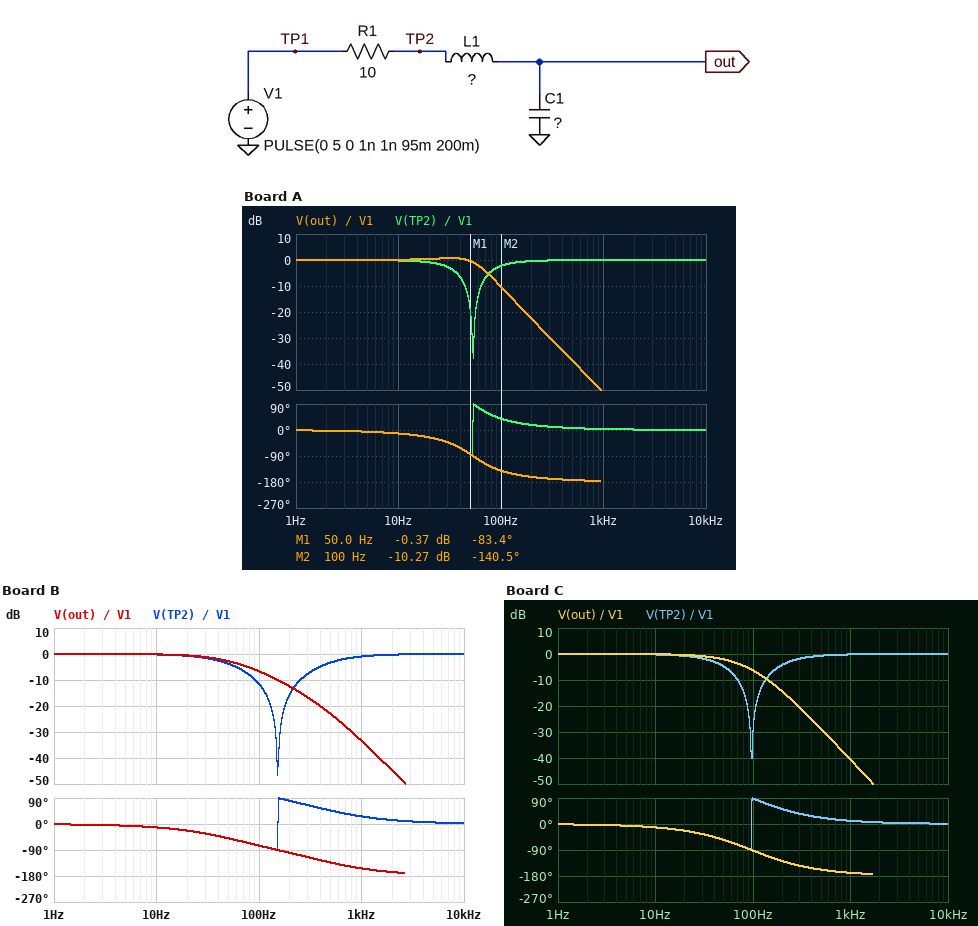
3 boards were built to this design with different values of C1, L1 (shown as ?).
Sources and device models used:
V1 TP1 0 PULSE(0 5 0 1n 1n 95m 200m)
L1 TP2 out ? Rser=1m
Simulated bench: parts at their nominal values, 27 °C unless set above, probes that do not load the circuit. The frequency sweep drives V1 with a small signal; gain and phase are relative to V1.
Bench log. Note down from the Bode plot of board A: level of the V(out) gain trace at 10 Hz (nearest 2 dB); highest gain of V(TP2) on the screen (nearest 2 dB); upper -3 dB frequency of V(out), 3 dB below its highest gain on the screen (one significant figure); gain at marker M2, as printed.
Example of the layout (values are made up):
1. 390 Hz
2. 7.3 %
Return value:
1. 0 dB
2. 0 dB
3. 60 Hz
4. -10.27 dB
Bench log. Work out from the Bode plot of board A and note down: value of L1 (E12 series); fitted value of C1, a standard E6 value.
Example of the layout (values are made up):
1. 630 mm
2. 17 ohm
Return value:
1. 27 mH
2. 330 µF
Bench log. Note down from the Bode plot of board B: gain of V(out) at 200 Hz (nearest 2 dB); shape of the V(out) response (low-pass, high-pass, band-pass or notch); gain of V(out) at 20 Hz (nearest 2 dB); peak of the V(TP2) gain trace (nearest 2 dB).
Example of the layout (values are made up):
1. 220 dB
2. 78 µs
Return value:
1. -12 dB
2. low-pass
3. 0 dB
4. 0 dB
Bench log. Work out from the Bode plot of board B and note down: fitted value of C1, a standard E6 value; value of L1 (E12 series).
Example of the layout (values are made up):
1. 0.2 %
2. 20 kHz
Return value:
1. 330 µF
2. 3.3 mH
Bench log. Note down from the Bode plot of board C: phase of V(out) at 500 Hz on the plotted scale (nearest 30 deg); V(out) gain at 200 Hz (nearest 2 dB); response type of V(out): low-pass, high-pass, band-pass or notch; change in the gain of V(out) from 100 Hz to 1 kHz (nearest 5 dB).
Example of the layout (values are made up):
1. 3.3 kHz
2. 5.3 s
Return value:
1. -150 deg
2. -14 dB
3. low-pass
4. -35 dB
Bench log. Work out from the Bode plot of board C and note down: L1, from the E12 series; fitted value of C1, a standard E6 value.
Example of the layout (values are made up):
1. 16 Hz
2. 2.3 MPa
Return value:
1. 8.2 mH
2. 330 µF
